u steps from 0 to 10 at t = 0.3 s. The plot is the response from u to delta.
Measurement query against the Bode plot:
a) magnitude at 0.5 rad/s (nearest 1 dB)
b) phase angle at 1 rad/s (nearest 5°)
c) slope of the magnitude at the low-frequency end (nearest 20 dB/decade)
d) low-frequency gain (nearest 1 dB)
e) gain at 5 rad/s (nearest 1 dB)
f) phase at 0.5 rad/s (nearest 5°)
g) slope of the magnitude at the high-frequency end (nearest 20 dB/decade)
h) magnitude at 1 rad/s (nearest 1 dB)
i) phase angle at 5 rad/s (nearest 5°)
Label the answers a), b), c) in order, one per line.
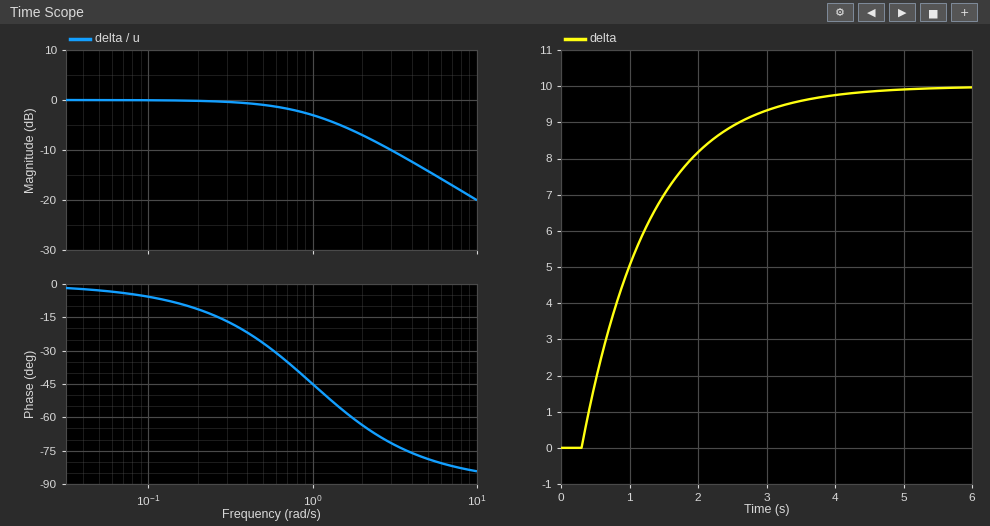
a) -1 dB
b) -45°
c) 0 dB/decade
d) 0 dB
e) -14 dB
f) -25°
g) -20 dB/decade
h) -3 dB
i) -80°
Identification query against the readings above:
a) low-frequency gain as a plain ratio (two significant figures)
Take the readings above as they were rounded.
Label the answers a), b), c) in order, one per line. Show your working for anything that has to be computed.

a) 10^(0 / 20) = 1.0
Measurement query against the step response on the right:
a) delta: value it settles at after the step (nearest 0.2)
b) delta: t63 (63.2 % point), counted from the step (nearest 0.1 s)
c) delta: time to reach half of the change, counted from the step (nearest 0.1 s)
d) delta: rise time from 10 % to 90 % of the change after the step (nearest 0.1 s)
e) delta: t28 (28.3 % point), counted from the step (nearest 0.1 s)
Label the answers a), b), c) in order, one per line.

a) 10.0
b) 1.0 s
c) 0.7 s
d) 2.2 s
e) 0.3 s
